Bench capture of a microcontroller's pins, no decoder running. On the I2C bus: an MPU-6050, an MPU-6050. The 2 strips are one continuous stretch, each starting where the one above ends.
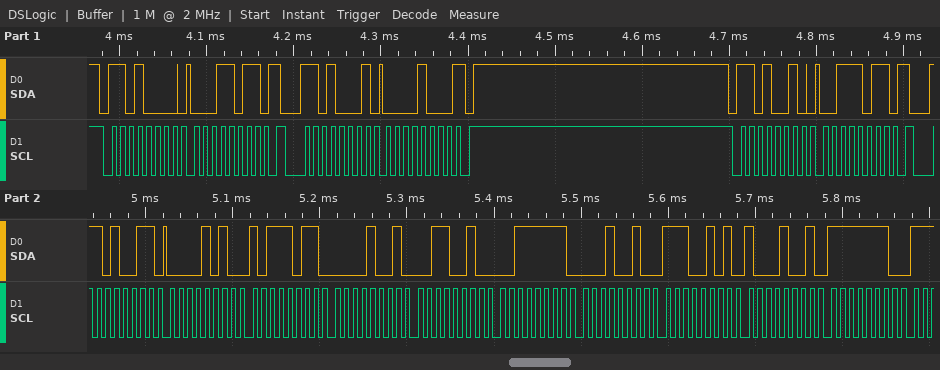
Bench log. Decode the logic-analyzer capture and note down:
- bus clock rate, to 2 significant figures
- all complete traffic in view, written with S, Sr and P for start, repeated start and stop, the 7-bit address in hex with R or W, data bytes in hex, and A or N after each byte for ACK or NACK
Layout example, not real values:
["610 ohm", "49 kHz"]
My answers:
["100 kHz", "S 68W A 1B A Sr 68R A 08 N P S 69W A 3B A Sr 69R A 0A A BB A 09 A 32 A 3F A 12 A E5 A 89 A FE A"]
